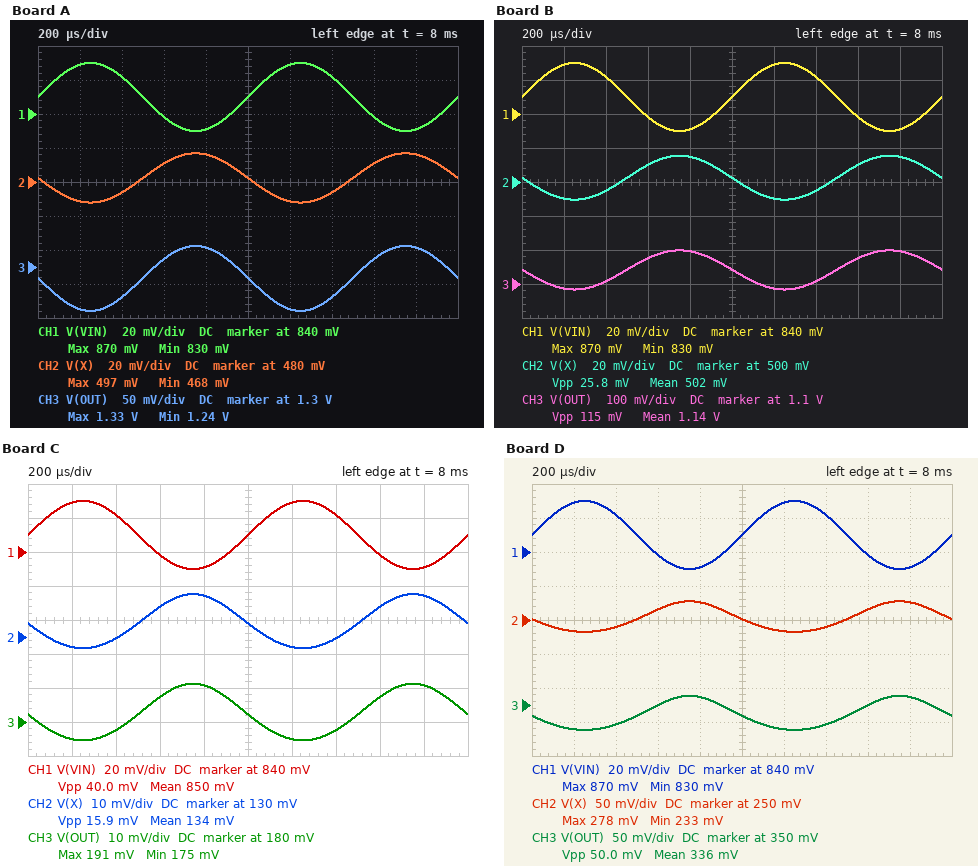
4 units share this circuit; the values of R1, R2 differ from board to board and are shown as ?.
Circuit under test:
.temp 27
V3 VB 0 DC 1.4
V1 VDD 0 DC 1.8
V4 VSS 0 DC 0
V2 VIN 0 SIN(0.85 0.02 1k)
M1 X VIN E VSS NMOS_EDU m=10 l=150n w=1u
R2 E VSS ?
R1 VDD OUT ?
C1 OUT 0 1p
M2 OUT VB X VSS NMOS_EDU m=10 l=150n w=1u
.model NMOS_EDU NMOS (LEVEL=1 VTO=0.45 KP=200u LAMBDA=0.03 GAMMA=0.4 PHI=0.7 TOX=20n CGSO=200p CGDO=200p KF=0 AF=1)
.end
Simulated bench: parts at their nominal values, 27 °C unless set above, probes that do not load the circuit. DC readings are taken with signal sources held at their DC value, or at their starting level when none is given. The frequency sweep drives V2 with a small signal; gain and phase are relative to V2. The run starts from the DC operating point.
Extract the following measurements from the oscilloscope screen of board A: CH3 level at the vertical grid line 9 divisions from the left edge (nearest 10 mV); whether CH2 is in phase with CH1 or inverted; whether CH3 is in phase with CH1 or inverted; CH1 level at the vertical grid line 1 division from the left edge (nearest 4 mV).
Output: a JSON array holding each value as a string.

["1.33 V", "inverted", "inverted", "868 mV"]
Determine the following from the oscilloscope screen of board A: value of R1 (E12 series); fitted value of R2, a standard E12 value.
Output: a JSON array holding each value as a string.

["560 Ω", "27 Ω"]
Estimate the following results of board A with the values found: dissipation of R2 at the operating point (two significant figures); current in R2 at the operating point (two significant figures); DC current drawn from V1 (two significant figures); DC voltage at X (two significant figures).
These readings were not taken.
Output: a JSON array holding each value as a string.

["23 µW", "920 µA", "920 µA", "480 mV"]
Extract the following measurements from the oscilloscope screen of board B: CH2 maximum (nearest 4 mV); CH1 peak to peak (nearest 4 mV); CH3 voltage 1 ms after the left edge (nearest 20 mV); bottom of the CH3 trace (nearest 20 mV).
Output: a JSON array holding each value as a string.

["516 mV", "40 mV", "1.14 V", "1.08 V"]
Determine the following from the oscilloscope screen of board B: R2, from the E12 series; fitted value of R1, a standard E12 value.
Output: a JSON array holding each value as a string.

["56 Ω", "820 Ω"]
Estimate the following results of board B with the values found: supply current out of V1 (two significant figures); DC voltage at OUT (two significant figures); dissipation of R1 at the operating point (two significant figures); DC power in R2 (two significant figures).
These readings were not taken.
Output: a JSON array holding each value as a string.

["800 µA", "1.1 V", "530 µW", "36 µW"]
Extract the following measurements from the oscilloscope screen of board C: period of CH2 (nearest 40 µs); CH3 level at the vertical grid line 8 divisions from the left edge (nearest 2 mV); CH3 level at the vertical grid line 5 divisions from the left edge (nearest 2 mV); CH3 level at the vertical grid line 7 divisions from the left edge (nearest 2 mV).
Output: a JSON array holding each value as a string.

["1.00 ms", "188 mV", "182 mV", "178 mV"]
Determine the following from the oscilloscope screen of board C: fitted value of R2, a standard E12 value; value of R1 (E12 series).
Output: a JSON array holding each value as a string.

["39 Ω", "3.3 kΩ"]
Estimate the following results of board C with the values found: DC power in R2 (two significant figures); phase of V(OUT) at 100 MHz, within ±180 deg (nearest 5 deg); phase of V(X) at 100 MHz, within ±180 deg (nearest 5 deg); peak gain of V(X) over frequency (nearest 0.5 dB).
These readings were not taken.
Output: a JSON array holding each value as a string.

["9.4 µW", "165 deg", "170 deg", "-8.0 dB"]
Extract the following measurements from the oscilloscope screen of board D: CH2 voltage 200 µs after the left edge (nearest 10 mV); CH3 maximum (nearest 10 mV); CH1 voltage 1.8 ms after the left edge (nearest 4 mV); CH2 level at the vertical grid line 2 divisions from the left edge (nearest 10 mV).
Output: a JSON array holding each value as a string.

["230 mV", "360 mV", "832 mV", "240 mV"]
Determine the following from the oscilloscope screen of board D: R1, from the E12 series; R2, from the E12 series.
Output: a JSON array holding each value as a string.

["2.2 kΩ", "68 Ω"]
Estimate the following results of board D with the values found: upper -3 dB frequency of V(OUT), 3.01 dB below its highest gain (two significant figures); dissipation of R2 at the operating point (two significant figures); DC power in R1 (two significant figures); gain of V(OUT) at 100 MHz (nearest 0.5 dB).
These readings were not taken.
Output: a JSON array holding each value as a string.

["230 MHz", "30 µW", "980 µW", "1.0 dB"]
